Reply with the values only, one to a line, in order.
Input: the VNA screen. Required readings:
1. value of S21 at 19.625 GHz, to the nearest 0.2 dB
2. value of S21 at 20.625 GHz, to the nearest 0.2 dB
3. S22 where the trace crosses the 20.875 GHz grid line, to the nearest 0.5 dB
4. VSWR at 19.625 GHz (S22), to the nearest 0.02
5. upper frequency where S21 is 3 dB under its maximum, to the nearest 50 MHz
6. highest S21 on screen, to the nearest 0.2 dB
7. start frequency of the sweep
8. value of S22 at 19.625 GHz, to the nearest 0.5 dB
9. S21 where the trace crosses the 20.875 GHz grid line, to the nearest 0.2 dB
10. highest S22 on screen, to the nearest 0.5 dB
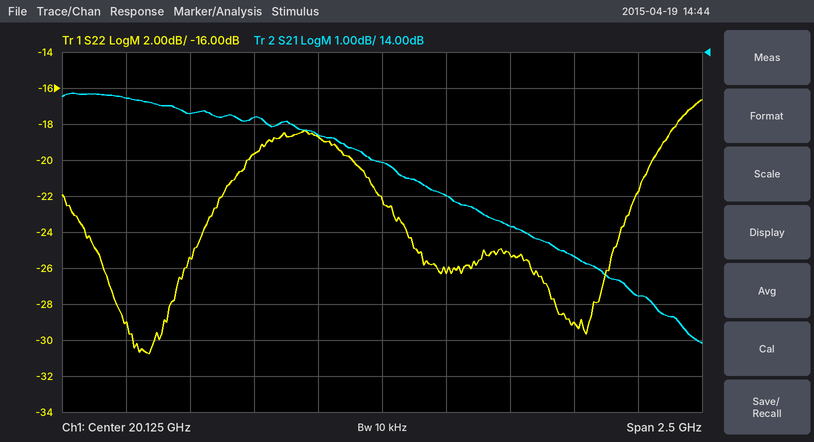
12.2 dB
9.2 dB
-29.0 dB
1.24
20.40 GHz
12.8 dB
18.875 GHz
-19.5 dB
8.4 dB
-16.5 dB
